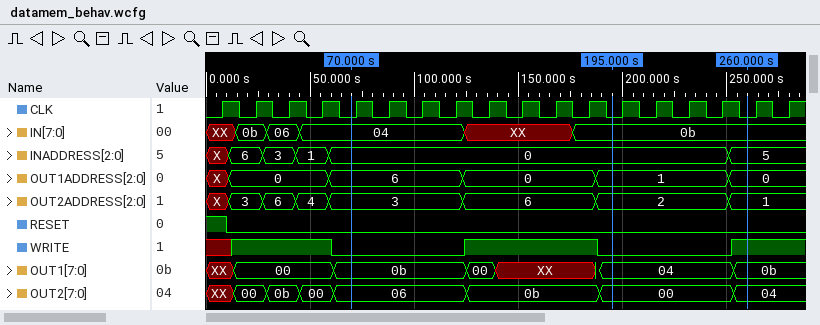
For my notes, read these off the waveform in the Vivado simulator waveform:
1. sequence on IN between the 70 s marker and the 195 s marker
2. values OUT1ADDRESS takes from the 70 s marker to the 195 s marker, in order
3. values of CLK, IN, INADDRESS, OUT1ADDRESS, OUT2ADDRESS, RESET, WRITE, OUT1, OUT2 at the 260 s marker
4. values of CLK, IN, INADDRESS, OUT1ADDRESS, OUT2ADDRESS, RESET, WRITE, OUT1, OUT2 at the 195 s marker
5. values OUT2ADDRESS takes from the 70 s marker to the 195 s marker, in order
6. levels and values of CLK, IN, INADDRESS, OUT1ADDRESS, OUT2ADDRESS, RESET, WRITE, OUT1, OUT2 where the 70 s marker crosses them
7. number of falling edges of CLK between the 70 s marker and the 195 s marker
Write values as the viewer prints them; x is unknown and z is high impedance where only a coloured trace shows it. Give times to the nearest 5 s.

04, XX, 0b
6, 0, 1
CLK=0, IN=0b, INADDRESS=5, OUT1ADDRESS=0, OUT2ADDRESS=1, RESET=0, WRITE=1, OUT1=0b, OUT2=04
CLK=0, IN=0b, INADDRESS=0, OUT1ADDRESS=1, OUT2ADDRESS=2, RESET=0, WRITE=0, OUT1=04, OUT2=00
3, 6, 2
CLK=0, IN=04, INADDRESS=0, OUT1ADDRESS=6, OUT2ADDRESS=3, RESET=0, WRITE=0, OUT1=0b, OUT2=06
8
